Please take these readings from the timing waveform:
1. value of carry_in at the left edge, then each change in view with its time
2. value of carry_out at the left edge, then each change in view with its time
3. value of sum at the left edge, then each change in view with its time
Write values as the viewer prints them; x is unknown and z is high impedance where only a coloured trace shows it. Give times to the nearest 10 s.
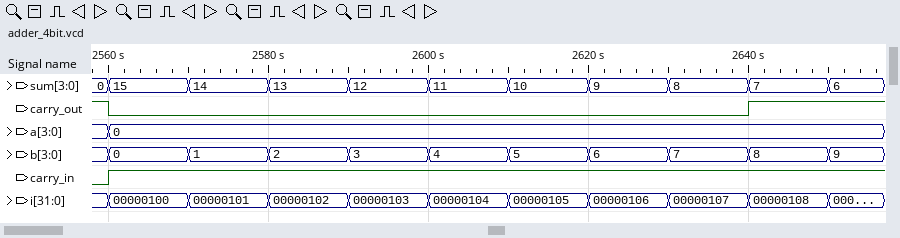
0, 1 at 2560 s
1, 0 at 2560 s, 1 at 2640 s
0, 15 at 2560 s, 14 at 2570 s, 13 at 2580 s, 12 at 2590 s, 11 at 2600 s, 10 at 2610 s, 9 at 2620 s, 8 at 2630 s, 7 at 2640 s, 6 at 2650 s
